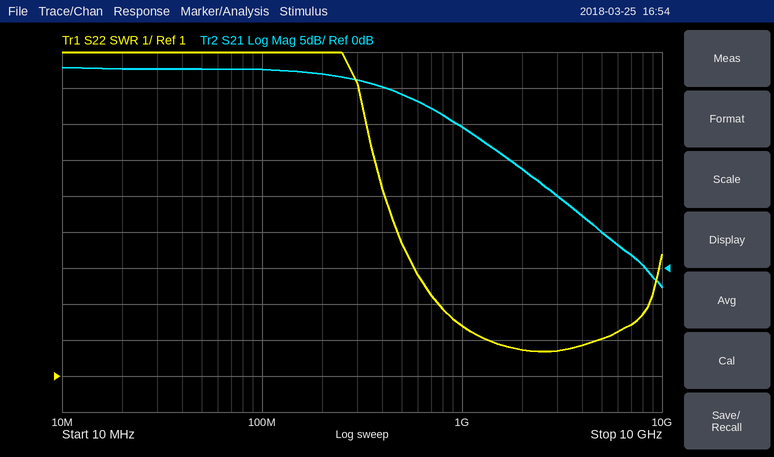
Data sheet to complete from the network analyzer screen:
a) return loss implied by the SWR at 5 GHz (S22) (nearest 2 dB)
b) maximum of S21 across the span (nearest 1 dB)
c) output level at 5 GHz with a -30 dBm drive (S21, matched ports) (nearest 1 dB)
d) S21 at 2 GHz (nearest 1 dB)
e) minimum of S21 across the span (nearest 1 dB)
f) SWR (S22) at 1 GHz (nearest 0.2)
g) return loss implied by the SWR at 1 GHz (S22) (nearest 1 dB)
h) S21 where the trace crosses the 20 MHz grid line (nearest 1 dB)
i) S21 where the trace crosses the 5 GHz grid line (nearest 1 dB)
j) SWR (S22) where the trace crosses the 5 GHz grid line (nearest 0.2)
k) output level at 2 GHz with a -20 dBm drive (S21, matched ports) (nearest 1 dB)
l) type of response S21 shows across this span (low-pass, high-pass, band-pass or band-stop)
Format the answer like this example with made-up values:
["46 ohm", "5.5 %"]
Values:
["10 dB", "28 dB", "-25 dBm", "14 dB", "-3 dB", "2.4", "8 dB", "28 dB", "5 dB", "2.0", "-6 dBm", "low-pass"]
